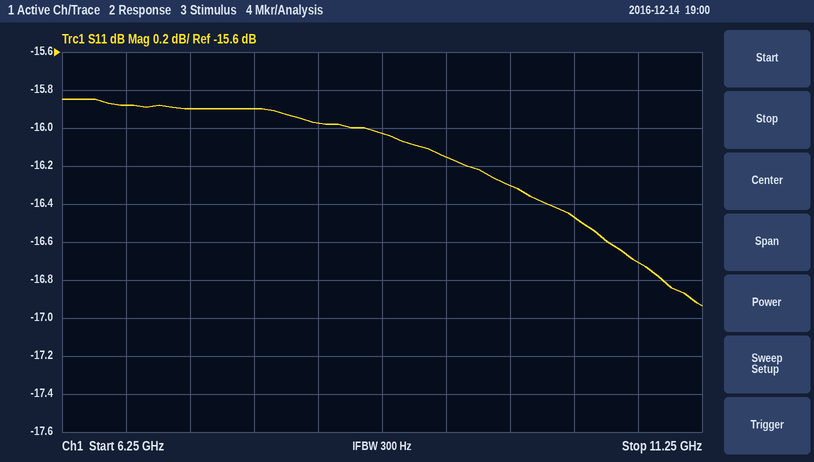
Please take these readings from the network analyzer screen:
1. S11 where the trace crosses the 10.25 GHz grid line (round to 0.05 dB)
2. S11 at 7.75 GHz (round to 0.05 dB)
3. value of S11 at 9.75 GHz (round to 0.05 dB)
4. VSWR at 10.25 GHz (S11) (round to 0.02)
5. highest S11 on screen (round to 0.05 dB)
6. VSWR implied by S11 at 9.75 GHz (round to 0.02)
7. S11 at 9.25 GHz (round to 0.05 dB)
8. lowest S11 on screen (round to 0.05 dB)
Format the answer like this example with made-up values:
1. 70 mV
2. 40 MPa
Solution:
1. -16.45 dB
2. -15.90 dB
3. -16.30 dB
4. 1.36
5. -15.85 dB
6. 1.36
7. -16.15 dB
8. -16.95 dB
